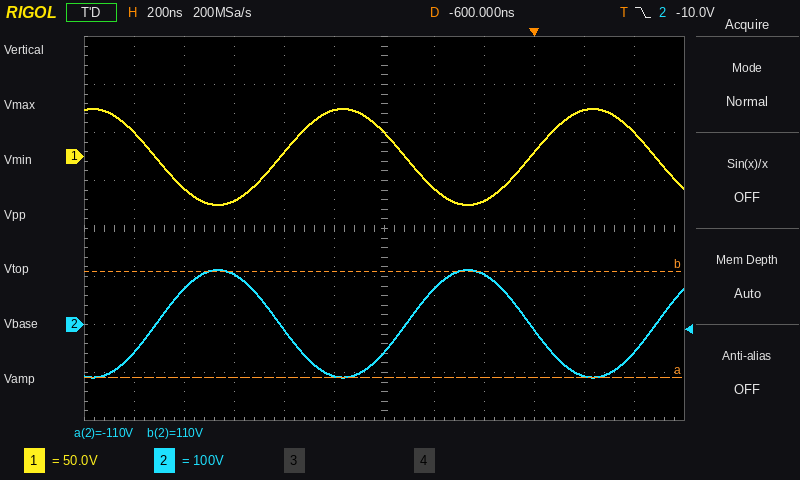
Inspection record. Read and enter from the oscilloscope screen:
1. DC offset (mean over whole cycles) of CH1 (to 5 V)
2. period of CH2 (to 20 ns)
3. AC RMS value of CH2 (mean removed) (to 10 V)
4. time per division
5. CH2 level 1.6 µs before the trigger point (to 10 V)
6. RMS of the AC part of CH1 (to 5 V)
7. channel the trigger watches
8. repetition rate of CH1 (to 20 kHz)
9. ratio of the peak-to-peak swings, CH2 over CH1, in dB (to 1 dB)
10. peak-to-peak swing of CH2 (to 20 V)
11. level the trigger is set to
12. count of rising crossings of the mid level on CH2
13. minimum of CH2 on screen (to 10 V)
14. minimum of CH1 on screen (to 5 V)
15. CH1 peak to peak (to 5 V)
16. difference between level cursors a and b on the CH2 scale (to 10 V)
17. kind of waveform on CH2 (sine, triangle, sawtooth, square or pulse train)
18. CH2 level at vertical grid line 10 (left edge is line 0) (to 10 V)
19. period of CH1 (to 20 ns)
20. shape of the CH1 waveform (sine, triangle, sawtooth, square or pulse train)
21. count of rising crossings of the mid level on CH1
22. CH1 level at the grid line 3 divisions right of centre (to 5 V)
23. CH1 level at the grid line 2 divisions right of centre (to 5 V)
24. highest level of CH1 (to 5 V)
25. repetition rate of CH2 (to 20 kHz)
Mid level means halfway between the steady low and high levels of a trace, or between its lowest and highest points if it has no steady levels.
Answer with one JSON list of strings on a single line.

["0 V", "1.00 µs", "80 V", "200 ns", "-60 V", "35 V", "CH2", "1.00 MHz", "7 dB", "220 V", "-10.0 V", "3", "-110 V", "-50 V", "100 V", "220 V", "sine", "-110 V", "1.00 µs", "sine", "2", "5 V", "-45 V", "50 V", "1.00 MHz"]
